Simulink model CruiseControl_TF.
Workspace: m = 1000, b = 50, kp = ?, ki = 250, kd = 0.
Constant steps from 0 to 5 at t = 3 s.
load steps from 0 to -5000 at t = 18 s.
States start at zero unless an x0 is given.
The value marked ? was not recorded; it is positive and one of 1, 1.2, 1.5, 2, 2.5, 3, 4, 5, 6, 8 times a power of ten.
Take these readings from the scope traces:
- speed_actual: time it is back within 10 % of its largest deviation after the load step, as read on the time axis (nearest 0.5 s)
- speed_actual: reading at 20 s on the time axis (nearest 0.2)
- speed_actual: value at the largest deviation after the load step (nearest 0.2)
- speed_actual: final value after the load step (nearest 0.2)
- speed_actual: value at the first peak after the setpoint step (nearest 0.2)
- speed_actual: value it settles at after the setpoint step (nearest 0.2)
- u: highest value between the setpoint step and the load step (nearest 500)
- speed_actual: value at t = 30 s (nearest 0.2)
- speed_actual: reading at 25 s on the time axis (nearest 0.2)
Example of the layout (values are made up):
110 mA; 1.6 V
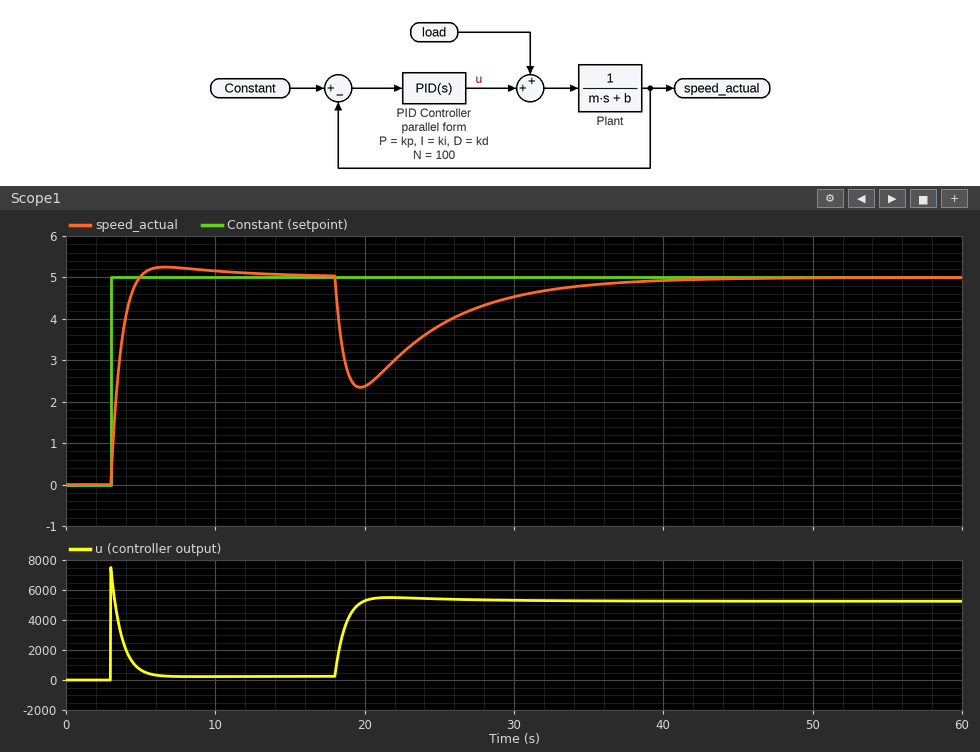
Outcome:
33.0 s; 2.4; 2.4; 5.0; 5.2; 5.0; 7500; 4.6; 3.8
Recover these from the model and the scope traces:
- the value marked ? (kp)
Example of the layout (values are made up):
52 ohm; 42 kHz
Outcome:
1500
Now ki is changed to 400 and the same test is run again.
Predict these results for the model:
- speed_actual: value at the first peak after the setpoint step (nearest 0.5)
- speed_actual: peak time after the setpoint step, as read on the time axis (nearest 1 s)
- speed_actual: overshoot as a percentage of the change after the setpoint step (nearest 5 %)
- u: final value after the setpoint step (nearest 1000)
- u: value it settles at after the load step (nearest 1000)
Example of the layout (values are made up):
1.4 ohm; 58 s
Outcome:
5.5; 6 s; 10 %; 0; 5000
